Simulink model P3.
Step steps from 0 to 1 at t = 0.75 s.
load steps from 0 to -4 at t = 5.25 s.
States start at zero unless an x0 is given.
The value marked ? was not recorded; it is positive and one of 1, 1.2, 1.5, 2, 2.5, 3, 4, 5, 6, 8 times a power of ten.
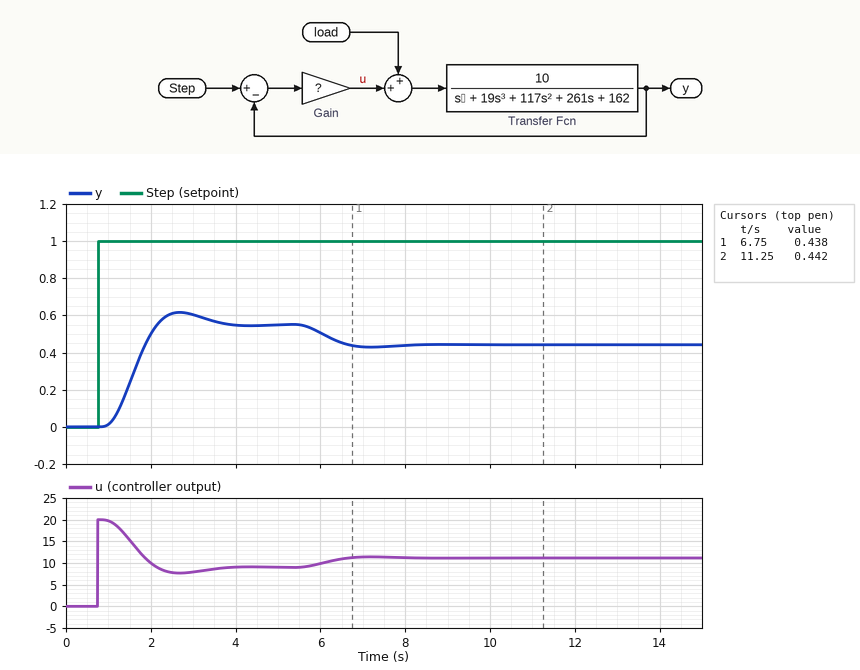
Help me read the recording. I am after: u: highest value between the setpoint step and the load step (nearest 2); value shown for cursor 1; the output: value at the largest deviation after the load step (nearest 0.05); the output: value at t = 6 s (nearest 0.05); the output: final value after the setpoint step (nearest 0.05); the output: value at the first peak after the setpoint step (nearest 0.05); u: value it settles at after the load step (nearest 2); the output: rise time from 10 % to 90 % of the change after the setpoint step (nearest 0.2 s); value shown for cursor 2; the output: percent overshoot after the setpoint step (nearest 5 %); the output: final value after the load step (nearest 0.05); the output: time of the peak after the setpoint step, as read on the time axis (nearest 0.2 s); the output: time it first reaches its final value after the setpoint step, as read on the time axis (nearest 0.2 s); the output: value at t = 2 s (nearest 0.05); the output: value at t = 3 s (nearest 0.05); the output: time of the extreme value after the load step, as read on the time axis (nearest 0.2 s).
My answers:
20
0.438
0.45
0.50
0.55
0.60
12
0.8 s
0.442
10 %
0.45
2.6 s
2.2 s
0.50
0.60
7.2 s
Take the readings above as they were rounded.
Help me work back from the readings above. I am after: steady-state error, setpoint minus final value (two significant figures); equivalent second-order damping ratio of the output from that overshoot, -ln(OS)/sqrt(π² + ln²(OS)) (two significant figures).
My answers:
0.45
0.59
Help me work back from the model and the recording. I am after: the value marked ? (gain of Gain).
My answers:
20
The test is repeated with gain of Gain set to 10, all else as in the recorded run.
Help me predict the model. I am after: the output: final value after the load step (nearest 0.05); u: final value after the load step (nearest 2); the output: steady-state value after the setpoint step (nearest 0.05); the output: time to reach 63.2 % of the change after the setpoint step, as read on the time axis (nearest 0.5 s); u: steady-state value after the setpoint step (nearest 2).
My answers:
0.25
8
0.40
2.0 s
6
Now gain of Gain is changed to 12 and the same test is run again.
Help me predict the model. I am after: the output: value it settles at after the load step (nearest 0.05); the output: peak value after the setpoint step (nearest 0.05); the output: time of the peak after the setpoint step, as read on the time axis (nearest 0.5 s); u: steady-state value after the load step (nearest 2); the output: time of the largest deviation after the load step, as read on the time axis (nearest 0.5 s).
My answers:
0.30
0.45
3.0 s
8
7.5 s
